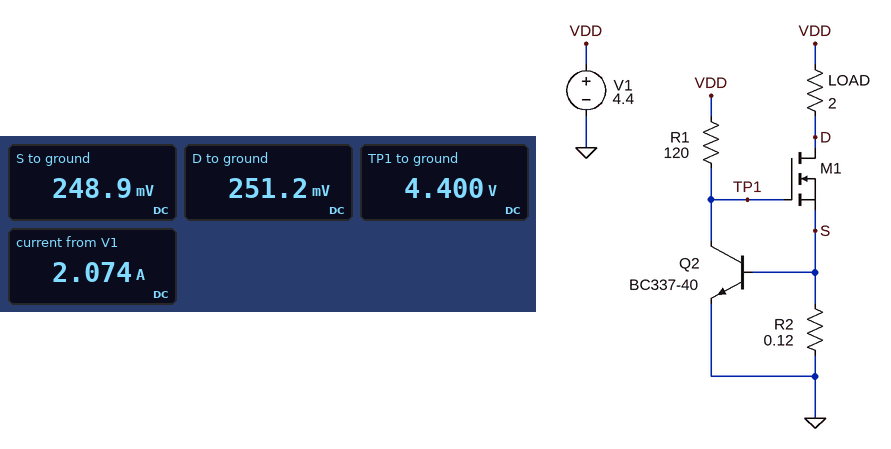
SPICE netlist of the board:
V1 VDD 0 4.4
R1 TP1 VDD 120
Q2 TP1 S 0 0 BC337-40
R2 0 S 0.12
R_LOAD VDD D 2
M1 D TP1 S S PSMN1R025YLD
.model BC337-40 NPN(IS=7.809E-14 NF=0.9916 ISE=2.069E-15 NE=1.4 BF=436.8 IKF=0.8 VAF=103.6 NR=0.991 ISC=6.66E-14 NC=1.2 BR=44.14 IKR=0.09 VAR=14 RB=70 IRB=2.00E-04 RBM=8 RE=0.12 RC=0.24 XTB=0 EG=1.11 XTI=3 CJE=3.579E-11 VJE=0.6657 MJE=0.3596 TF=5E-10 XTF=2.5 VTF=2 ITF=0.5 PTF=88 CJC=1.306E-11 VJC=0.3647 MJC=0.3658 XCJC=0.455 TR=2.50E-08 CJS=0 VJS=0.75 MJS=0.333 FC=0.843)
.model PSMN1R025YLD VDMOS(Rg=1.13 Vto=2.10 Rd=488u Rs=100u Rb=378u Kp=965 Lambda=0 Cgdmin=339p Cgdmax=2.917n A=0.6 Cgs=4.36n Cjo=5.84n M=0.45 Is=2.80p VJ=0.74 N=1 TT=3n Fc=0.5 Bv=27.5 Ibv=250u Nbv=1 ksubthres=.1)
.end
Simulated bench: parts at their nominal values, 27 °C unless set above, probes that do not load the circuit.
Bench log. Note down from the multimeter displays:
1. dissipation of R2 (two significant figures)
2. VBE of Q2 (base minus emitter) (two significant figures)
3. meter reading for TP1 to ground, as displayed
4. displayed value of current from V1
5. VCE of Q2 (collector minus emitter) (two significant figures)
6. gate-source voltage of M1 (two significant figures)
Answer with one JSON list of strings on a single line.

["520 mW", "250 mV", "4.400 V", "2.074 A", "4.4 V", "4.2 V"]
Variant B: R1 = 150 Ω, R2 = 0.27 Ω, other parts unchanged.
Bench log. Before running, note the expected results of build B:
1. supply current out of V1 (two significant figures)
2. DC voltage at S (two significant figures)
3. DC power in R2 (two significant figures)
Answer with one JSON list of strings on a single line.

["1.9 A", "520 mV", "1.0 W"]
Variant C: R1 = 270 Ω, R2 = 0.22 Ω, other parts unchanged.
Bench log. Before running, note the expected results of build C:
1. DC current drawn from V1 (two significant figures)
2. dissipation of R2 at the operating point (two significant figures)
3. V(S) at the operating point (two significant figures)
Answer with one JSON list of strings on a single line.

["2.0 A", "860 mW", "440 mV"]
